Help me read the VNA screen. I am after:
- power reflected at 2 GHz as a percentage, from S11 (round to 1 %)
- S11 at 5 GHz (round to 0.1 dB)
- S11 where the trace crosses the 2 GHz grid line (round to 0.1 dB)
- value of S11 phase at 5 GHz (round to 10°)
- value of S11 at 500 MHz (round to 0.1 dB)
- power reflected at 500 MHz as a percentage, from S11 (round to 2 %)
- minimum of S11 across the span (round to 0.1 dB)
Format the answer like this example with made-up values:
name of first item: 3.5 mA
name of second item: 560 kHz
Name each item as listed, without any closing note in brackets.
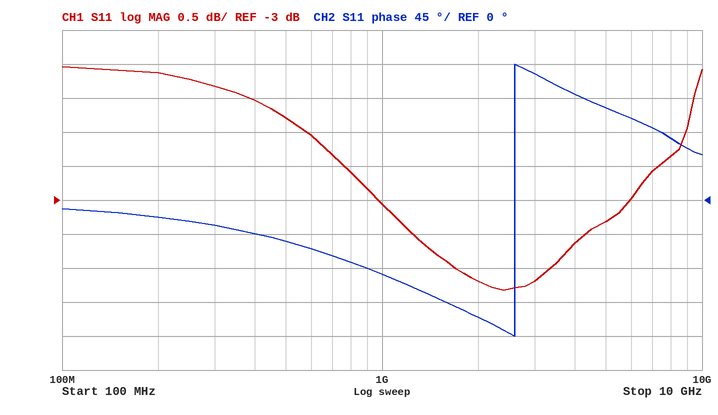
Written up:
power reflected at 2 GHz as a percentage, from S11: 38 %
S11 at 5 GHz: -3.3 dB
S11 where the trace crosses the 2 GHz grid line: -4.2 dB
value of S11 phase at 5 GHz: 120°
value of S11 at 500 MHz: -1.8 dB
power reflected at 500 MHz as a percentage, from S11: 66 %
minimum of S11 across the span: -4.3 dB
